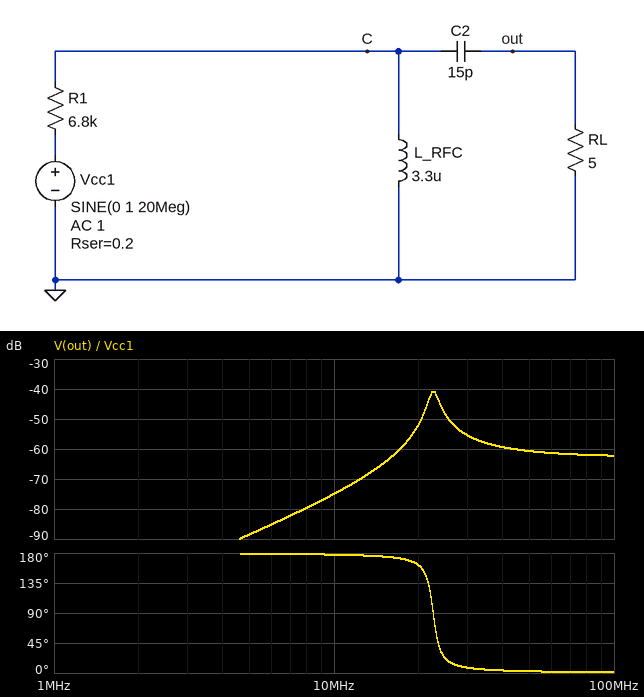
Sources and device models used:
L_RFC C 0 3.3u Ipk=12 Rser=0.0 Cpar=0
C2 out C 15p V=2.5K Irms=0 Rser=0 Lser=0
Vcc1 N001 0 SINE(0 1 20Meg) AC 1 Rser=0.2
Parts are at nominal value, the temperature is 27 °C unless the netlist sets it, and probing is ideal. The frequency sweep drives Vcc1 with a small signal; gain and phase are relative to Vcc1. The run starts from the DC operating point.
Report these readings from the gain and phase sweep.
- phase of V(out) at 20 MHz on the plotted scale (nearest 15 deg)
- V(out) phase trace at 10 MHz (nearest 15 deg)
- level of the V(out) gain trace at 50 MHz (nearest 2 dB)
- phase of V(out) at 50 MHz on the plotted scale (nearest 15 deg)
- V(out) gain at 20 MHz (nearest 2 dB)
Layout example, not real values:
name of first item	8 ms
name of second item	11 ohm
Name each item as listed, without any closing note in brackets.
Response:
phase of V(out) at 20 MHz on the plotted scale	165 deg
V(out) phase trace at 10 MHz	180 deg
level of the V(out) gain trace at 50 MHz	-60 dB
phase of V(out) at 50 MHz on the plotted scale	0 deg
V(out) gain at 20 MHz	-52 dB
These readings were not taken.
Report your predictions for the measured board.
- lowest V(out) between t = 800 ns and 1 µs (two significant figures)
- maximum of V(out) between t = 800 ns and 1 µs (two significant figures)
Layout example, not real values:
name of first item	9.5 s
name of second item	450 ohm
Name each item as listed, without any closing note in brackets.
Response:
lowest V(out) between t = 800 ns and 1 µs	-2.5 mV
maximum of V(out) between t = 800 ns and 1 µs	2.5 mV
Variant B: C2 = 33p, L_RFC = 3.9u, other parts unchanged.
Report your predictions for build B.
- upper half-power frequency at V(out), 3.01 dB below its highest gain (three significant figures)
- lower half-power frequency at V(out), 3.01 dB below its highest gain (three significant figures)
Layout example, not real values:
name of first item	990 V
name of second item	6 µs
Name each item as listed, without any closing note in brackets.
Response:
upper half-power frequency at V(out), 3.01 dB below its highest gain	14.5 MHz
lower half-power frequency at V(out), 3.01 dB below its highest gain	13.6 MHz
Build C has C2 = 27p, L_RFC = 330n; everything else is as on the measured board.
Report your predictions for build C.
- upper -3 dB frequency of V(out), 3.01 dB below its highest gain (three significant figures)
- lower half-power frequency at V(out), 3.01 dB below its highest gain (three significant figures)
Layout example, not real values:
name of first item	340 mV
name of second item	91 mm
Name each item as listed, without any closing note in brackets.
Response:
upper -3 dB frequency of V(out), 3.01 dB below its highest gain	55.1 MHz
lower half-power frequency at V(out), 3.01 dB below its highest gain	51.8 MHz
